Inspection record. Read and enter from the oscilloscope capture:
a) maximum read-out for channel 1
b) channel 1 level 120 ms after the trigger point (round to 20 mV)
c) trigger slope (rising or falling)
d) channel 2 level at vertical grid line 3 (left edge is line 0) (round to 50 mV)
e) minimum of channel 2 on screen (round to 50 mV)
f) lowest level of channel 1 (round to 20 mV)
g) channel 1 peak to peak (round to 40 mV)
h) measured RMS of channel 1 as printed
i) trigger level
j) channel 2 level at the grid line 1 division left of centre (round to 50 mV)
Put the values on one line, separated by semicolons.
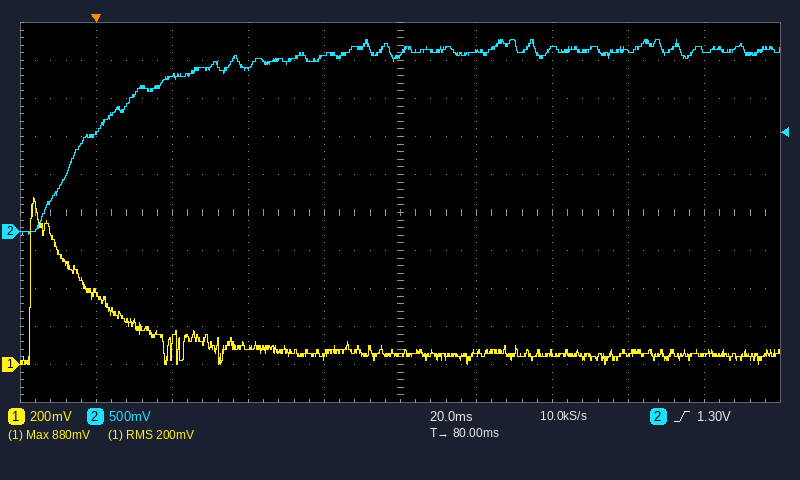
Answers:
880 mV; 60 mV; rising; 2.15 V; -50 mV; 0 mV; 880 mV; 200 mV; 1.30 V; 2.30 V
